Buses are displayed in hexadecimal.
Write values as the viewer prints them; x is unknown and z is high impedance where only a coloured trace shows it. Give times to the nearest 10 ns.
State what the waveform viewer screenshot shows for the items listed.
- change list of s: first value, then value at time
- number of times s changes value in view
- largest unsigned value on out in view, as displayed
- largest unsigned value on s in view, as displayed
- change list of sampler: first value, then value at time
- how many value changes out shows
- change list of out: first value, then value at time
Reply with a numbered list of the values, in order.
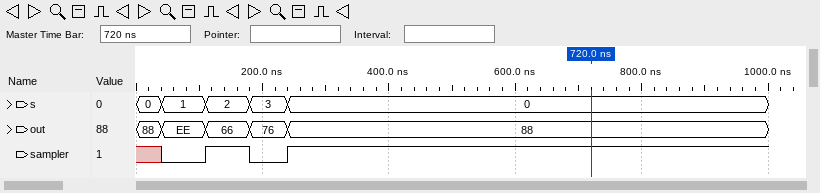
1. 0, 1 at 40 ns, 2 at 110 ns, 3 at 180 ns, 0 at 240 ns
2. 4
3. EE
4. 3
5. x, 0 at 40 ns, 1 at 110 ns, 0 at 180 ns, 1 at 240 ns
6. 4
7. 88, EE at 40 ns, 66 at 110 ns, 76 at 180 ns, 88 at 240 ns
